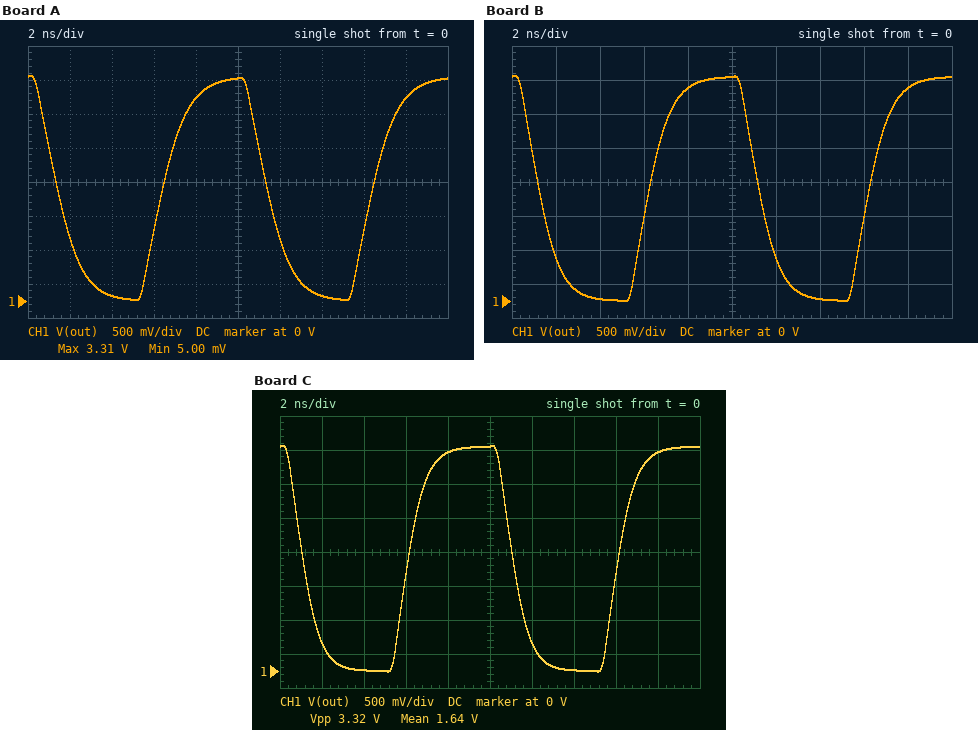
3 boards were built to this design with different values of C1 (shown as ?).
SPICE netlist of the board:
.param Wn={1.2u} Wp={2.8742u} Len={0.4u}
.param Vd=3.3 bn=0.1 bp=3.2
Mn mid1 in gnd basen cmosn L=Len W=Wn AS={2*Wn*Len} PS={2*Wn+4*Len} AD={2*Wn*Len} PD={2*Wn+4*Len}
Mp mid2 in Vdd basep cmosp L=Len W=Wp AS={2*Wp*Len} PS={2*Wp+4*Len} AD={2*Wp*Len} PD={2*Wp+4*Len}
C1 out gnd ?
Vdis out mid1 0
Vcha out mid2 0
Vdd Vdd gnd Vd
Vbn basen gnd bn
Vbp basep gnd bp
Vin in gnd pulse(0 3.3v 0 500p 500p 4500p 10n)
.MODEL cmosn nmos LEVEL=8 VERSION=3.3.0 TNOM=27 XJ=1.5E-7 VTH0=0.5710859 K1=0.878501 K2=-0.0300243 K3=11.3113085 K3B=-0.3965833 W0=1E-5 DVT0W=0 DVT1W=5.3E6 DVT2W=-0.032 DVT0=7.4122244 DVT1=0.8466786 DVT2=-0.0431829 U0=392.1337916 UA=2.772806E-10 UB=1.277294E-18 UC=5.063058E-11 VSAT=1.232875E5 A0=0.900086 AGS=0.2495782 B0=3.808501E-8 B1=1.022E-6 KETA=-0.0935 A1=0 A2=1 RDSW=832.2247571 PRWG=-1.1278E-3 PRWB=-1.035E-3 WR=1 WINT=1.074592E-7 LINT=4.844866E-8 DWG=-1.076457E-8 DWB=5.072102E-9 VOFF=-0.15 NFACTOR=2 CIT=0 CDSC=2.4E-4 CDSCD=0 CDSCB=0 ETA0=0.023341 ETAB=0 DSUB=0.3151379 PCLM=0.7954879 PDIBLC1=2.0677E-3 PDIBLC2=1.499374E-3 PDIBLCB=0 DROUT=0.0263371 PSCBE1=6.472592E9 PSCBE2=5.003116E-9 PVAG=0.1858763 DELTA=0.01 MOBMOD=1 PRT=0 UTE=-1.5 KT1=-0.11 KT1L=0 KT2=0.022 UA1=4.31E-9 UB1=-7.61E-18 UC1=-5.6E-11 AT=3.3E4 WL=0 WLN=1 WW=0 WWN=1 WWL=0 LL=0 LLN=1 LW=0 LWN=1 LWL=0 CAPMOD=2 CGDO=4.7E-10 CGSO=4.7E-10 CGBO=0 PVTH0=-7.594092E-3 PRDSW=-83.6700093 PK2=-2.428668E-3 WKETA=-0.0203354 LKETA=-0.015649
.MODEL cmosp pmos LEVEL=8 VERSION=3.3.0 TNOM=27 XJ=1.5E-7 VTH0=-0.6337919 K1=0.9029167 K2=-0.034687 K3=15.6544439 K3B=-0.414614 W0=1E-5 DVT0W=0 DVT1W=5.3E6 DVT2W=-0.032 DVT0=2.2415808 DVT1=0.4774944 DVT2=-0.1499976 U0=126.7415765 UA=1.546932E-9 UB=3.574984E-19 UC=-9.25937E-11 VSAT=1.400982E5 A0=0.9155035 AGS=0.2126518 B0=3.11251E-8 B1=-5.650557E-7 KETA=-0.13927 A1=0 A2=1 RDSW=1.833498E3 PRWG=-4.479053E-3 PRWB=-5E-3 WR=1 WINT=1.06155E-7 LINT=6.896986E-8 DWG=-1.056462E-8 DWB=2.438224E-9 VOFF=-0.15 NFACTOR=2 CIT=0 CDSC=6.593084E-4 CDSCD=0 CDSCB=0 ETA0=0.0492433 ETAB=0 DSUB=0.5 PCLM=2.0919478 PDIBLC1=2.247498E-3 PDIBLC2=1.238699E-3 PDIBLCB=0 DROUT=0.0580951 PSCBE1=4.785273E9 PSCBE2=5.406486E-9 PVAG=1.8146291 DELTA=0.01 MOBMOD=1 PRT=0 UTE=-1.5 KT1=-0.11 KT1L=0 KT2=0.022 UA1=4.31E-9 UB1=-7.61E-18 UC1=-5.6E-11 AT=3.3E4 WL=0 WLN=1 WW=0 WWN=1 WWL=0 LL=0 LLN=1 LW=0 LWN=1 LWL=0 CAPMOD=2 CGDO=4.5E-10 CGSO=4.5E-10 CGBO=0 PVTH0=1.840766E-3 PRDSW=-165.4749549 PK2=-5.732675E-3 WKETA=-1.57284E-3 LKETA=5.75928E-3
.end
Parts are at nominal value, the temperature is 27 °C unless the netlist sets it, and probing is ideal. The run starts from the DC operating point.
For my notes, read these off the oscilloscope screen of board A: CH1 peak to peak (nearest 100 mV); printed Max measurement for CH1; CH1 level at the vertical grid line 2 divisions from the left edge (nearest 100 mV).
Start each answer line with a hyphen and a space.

- 3.3 V
- 3.31 V
- 100 mV
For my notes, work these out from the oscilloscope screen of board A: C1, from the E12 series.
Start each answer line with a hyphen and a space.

- 470 fF
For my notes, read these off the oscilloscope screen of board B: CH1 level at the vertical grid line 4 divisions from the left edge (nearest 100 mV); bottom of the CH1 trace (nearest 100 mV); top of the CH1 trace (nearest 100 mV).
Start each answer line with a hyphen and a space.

- 3.1 V
- 0 V
- 3.3 V
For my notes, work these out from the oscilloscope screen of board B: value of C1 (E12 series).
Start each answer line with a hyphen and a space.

- 390 fF
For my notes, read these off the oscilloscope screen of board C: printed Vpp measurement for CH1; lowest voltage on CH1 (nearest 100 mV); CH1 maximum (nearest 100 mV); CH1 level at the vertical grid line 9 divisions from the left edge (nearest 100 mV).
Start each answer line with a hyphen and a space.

- 3.32 V
- 0 V
- 3.3 V
- 3.2 V
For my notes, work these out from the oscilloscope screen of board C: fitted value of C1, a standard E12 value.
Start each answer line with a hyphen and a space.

- 330 fF
